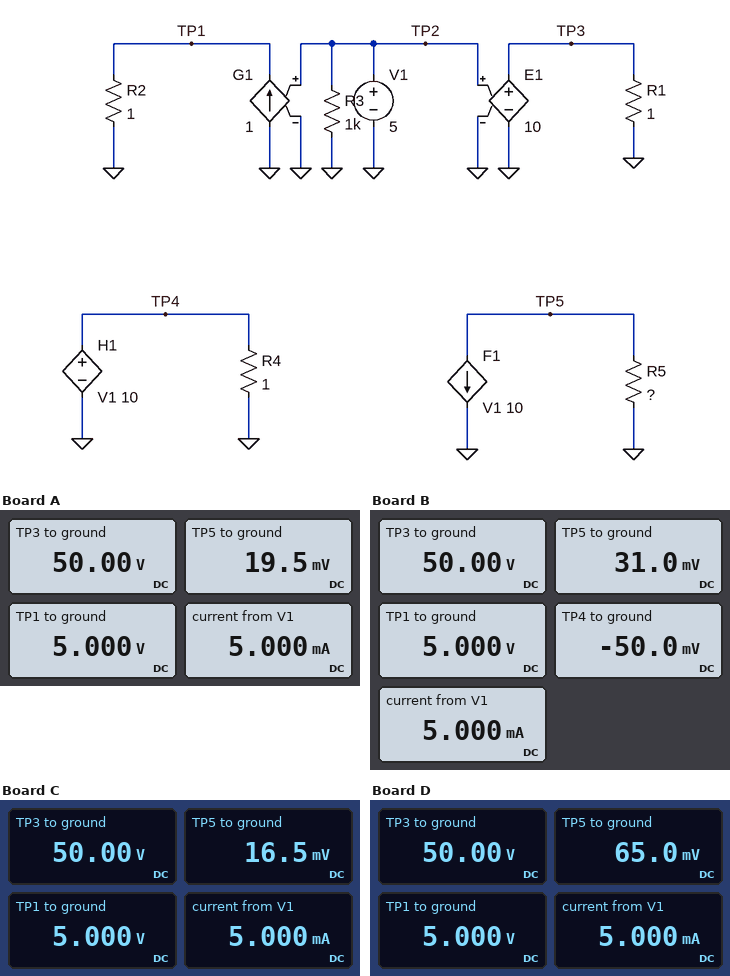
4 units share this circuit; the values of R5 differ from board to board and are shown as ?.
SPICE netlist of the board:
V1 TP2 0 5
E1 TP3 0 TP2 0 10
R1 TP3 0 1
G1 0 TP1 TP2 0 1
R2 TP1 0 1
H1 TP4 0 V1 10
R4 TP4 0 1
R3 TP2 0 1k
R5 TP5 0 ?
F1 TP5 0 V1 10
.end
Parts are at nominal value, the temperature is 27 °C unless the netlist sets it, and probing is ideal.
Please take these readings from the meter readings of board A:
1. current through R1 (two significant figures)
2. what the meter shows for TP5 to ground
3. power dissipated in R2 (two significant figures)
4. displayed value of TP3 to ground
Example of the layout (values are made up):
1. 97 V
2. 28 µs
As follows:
1. 50 A
2. 19.5 mV
3. 25 W
4. 50.00 V
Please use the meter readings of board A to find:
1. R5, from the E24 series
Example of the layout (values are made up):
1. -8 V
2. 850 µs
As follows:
1. 0.39 Ω
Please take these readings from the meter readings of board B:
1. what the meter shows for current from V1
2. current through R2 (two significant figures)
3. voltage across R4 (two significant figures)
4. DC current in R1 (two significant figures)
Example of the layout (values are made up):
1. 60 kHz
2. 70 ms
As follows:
1. 5.000 mA
2. 5.0 A
3. 50 mV
4. 50 A
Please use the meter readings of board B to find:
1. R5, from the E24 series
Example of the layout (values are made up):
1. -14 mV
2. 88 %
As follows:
1. 0.62 Ω
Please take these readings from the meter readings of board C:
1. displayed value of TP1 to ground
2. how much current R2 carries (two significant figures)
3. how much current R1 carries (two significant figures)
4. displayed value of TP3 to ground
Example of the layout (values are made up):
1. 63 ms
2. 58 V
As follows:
1. 5.000 V
2. 5.0 A
3. 50 A
4. 50.00 V
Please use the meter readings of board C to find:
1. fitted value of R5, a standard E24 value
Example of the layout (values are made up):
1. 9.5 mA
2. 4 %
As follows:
1. 0.33 Ω
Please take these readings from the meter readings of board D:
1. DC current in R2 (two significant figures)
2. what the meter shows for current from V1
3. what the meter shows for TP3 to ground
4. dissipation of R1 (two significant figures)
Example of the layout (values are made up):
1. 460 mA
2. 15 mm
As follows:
1. 5.0 A
2. 5.000 mA
3. 50.00 V
4. 2.5 kW
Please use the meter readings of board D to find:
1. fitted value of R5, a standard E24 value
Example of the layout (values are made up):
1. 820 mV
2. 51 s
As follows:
1. 1.3 Ω
